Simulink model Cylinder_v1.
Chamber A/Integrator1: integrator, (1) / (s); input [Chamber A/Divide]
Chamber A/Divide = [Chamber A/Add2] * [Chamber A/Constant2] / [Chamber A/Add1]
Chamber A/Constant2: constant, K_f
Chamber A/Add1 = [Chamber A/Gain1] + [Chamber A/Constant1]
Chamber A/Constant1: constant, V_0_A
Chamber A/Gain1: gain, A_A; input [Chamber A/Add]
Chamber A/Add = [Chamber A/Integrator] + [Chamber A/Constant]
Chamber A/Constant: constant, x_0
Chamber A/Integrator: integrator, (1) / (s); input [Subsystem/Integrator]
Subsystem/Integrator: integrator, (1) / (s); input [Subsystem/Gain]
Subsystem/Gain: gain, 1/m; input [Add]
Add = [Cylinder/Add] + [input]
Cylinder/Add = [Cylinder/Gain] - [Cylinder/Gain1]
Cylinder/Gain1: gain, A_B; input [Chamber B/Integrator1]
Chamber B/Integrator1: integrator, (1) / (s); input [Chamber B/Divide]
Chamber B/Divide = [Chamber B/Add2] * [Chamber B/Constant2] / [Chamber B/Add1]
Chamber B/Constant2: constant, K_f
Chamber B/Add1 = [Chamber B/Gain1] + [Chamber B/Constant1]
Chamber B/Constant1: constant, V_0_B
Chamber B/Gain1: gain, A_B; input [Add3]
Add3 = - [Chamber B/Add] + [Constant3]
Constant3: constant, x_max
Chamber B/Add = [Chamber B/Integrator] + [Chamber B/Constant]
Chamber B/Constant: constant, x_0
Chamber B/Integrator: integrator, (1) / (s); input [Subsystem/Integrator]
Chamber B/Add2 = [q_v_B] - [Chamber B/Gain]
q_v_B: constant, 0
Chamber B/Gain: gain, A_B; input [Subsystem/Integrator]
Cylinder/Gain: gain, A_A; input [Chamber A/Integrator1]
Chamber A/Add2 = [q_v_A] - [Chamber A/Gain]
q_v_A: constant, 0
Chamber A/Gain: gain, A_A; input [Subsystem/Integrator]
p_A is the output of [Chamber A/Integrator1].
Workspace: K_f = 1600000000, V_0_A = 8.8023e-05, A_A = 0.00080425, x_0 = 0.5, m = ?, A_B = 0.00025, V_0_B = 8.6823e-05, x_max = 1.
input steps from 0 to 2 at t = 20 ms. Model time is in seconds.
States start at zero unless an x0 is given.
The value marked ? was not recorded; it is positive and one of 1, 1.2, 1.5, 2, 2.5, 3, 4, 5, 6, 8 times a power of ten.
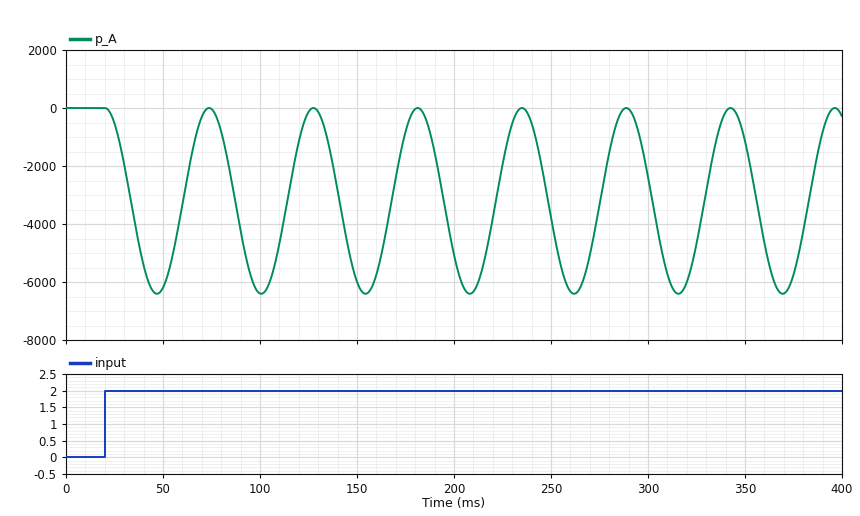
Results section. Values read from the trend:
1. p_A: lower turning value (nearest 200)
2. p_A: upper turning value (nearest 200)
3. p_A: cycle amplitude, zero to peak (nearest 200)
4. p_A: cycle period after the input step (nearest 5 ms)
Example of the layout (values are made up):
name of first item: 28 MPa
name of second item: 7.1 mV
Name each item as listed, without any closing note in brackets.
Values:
p_A: lower turning value: -6400
p_A: upper turning value: 0
p_A: cycle amplitude, zero to peak: 3200
p_A: cycle period after the input step: 55 ms
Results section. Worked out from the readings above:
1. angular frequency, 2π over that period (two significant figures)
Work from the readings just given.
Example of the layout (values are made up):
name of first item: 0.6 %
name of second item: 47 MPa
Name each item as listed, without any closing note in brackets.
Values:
angular frequency, 2π over that period: 0.11 rad/ms
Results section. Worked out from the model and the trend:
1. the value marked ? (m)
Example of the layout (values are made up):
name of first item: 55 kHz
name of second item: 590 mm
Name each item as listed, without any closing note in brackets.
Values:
the value marked ?: 120
